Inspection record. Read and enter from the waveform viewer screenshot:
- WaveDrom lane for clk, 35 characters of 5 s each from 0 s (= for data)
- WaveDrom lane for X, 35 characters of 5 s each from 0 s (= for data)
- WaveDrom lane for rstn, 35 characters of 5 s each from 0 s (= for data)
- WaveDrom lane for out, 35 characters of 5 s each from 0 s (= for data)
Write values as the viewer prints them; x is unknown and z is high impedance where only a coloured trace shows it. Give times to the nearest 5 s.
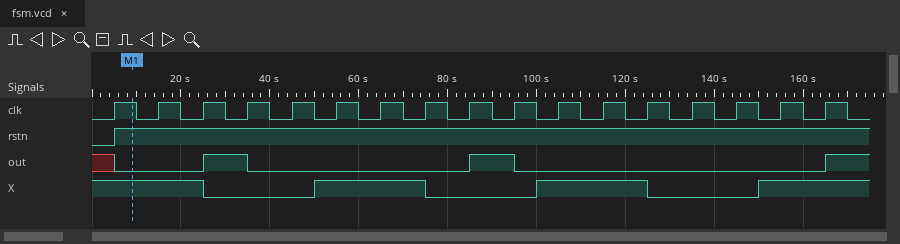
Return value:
{name: 'clk', wave: '01010101010101010101010101010101010'}
{name: 'X', wave: '1....0....1....0....1....0....1....'}
{name: 'rstn', wave: '01.................................'}
{name: 'out', wave: 'x0...1.0.........1.0.............1.'}
